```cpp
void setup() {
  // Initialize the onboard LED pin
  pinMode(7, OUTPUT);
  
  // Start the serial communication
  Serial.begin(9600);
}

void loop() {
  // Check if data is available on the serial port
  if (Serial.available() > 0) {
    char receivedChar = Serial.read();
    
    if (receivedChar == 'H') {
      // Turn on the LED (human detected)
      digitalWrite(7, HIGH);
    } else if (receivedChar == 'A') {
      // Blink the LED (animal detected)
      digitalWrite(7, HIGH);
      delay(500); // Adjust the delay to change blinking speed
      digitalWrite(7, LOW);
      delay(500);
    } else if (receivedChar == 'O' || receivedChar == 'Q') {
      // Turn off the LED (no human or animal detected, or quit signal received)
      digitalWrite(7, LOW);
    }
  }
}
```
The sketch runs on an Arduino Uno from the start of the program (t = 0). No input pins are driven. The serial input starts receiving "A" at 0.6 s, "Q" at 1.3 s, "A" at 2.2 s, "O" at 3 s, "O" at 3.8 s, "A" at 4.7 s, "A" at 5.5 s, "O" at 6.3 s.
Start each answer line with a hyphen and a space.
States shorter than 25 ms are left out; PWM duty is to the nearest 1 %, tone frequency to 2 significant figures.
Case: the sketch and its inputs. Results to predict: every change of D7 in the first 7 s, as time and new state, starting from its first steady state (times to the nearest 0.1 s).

- 0 s low; 0.6 s high; 1.1 s low; 2.2 s high; 2.7 s low; 4.7 s high; 5.2 s low; 5.7 s high; 6.2 s low
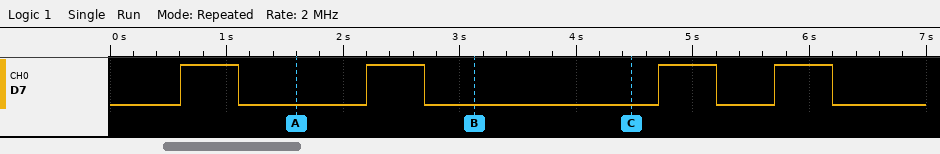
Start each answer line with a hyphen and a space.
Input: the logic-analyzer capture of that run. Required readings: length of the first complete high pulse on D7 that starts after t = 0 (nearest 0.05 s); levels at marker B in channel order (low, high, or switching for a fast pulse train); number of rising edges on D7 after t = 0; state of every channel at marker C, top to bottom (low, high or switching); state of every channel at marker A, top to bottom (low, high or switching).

- 0.50 s
- D7 low
- 4
- D7 low
- D7 low
